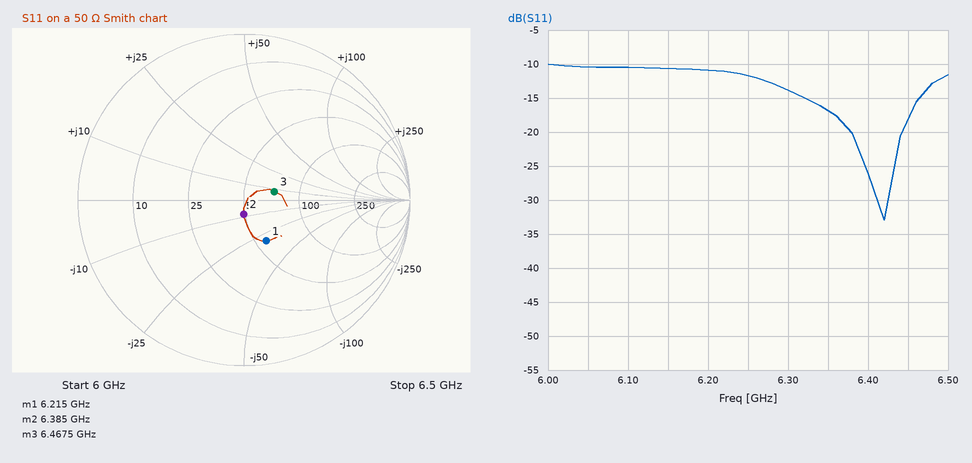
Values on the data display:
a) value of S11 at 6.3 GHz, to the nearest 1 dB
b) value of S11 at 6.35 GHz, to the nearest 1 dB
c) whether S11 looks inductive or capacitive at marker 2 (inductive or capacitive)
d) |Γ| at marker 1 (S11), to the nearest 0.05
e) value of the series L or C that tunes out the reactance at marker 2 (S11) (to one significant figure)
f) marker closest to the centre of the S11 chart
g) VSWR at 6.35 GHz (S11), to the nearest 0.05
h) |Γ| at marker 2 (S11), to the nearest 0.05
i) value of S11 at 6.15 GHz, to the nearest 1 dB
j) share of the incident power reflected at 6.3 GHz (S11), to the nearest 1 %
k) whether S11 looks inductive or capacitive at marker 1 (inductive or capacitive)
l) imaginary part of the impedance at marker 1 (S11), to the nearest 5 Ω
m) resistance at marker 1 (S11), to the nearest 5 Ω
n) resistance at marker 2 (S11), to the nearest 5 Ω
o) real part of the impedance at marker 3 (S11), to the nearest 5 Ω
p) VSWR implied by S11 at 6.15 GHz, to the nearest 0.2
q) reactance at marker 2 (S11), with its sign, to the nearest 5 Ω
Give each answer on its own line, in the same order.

-14 dB
-17 dB
capacitive
0.30
200 pH
marker 2
1.35
0.10
-11 dB
4 %
capacitive
-30 Ω
55 Ω
50 Ω
70 Ω
1.8
-10 Ω
